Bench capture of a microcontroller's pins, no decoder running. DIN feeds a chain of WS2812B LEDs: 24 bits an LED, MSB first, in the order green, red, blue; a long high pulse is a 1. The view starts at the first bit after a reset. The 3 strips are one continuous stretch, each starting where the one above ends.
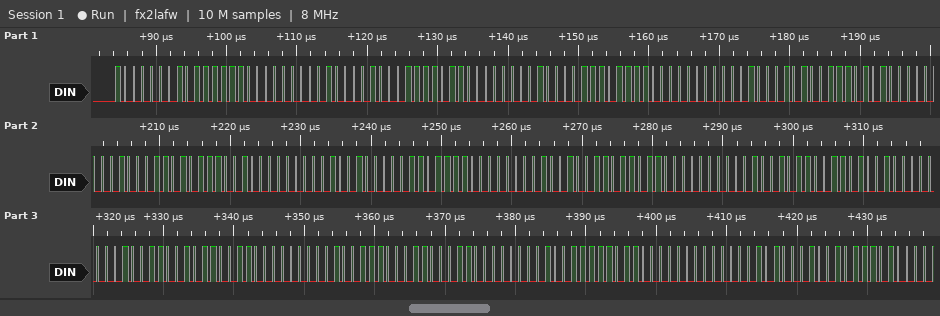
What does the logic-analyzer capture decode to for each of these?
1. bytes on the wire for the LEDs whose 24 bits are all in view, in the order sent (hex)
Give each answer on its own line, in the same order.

81 7E 00 84 7B 00 87 78 00 8A 75 00 8D 72 00 90 6F 00 93 6C 00 96 69 00 99 66 00 9C 63 00 9F 60 00
